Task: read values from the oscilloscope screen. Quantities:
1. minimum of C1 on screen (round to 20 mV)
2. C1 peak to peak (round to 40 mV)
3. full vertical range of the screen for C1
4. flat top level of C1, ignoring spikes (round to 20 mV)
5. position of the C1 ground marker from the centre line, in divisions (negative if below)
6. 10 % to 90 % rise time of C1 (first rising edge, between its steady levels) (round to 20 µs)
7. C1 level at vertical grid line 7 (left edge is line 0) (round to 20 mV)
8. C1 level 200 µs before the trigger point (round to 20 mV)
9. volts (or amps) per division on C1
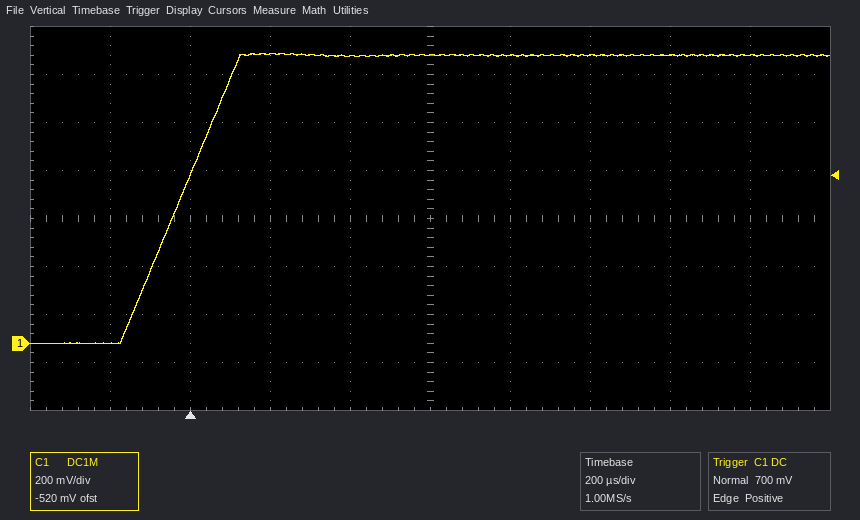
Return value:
0 mV
1.20 V
1.6 V
1.20 V
-2.6 div
240 µs
1.20 V
0 mV
200 mV
